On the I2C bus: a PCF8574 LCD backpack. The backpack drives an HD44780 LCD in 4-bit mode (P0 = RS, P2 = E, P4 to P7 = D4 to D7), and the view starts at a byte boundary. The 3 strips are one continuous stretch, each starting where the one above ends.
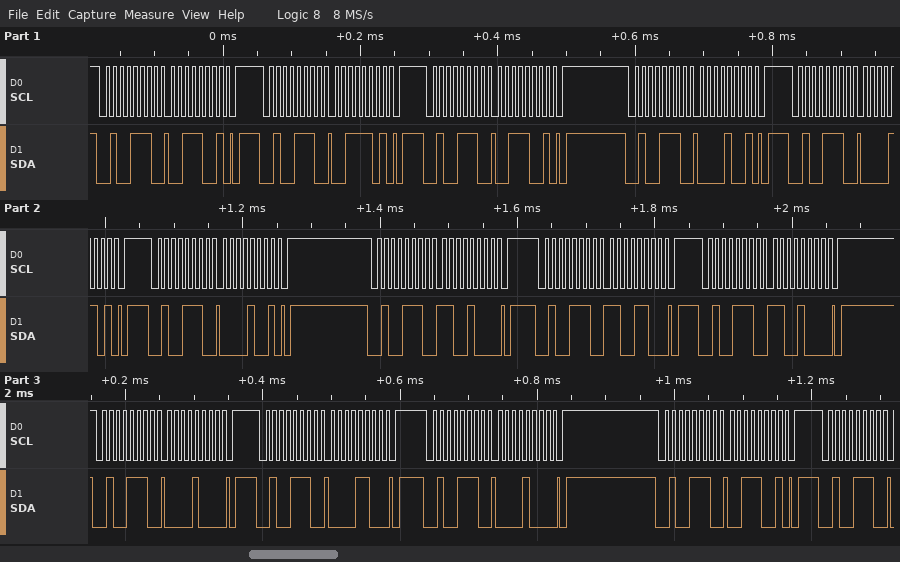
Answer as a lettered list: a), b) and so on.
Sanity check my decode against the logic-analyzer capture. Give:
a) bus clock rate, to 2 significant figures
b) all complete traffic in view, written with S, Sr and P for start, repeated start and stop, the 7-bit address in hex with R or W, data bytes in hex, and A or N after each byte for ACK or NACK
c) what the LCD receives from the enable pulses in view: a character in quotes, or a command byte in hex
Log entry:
a) 100 kHz
b) S 27W A 39 A P S 27W A 3D A P S 27W A 39 A P S 27W A 09 A P S 27W A 0D A P S 27W A 09 A P S 27W A C8 A P S 27W A CC A P S 27W A C8 A P S 27W A 08 A P S 27W A 0C A P S 27W A 08 A P S 27W A 39 A P S 27W A
c) '0' 0xC0
